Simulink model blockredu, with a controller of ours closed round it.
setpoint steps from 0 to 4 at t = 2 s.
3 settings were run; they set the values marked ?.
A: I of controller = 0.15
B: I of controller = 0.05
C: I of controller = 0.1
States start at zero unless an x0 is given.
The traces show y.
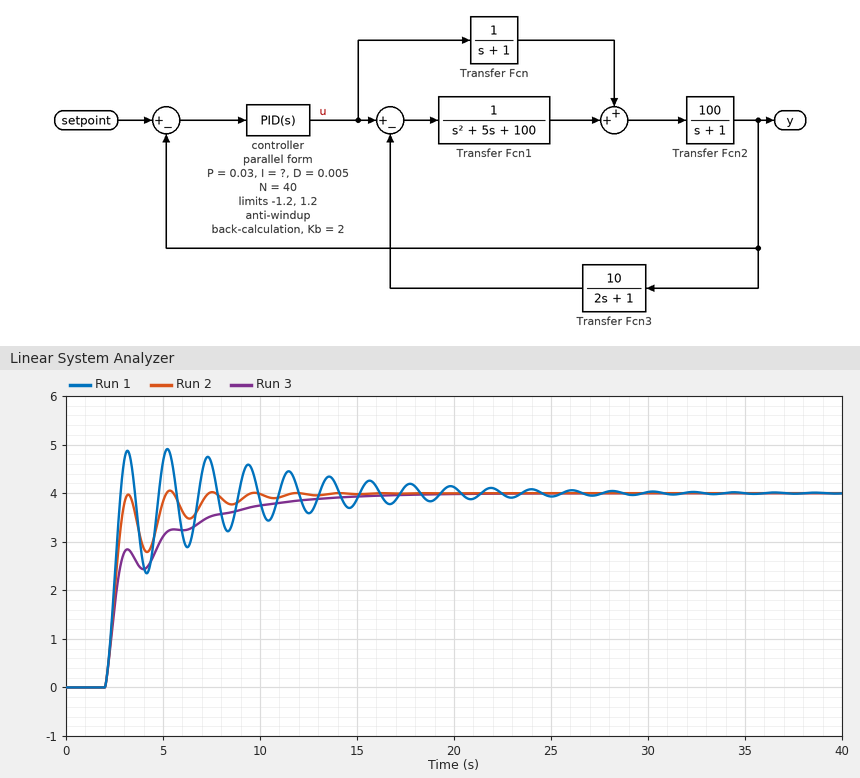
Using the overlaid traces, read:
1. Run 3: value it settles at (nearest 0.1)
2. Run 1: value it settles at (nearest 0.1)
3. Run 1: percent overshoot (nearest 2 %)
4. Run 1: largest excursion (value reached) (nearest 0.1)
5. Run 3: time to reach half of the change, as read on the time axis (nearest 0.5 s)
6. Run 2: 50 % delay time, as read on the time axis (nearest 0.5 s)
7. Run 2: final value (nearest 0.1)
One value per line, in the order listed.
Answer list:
4.0
4.0
22 %
4.9
2.5 s
2.5 s
4.0
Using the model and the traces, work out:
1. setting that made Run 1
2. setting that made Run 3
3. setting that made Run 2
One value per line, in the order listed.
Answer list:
A
B
C
